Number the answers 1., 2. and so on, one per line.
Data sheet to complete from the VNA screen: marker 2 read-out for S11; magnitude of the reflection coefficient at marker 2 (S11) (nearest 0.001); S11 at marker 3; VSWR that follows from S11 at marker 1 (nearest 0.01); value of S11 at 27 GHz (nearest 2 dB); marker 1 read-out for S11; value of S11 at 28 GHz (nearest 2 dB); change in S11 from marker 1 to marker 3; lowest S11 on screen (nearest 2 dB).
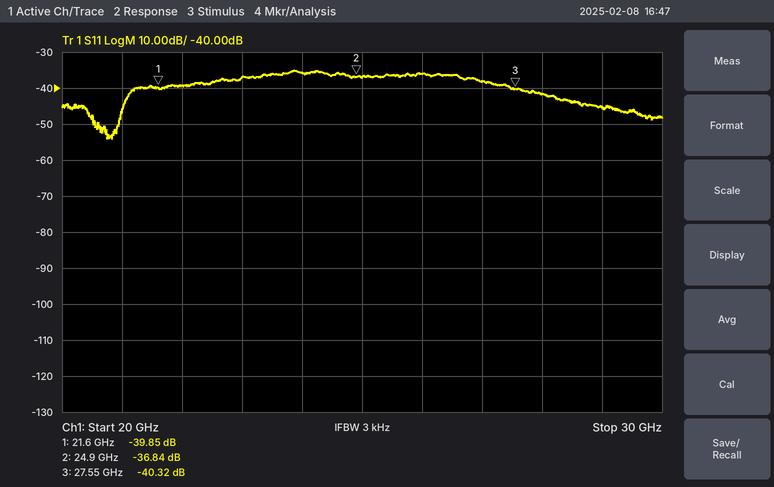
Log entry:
1. -36.84 dB
2. 0.014
3. -40.32 dB
4. 1.02
5. -38 dB
6. -39.85 dB
7. -42 dB
8. -0.47 dB
9. -54 dB
